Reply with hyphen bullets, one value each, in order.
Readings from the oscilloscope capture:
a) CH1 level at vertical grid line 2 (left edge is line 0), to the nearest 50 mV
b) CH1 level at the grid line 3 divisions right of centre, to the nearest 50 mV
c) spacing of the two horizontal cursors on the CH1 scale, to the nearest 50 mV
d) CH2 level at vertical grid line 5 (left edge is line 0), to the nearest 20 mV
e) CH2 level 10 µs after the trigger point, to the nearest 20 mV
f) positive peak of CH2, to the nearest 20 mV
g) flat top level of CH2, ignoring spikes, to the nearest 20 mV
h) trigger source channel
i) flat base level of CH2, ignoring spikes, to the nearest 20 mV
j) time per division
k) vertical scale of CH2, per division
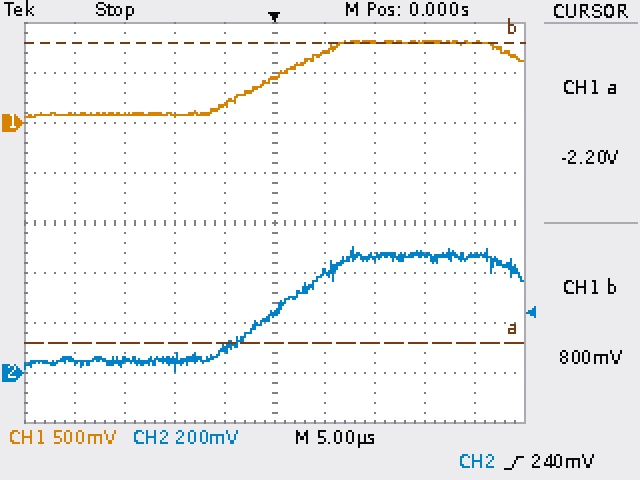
- 100 mV
- 800 mV
- 3.00 V
- 240 mV
- 460 mV
- 500 mV
- 460 mV
- CH2
- 40 mV
- 5 µs
- 200 mV
